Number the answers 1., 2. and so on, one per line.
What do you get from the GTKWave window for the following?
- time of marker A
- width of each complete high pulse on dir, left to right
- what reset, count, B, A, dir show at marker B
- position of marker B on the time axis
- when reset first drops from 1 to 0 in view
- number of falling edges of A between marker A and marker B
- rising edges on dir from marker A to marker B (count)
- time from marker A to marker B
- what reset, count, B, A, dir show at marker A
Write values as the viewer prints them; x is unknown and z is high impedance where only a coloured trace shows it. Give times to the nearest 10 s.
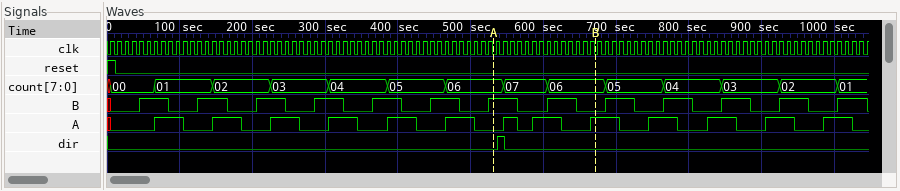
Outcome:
1. 530 s
2. 10 s
3. reset=0, count=06, B=0, A=1, dir=0
4. 670 s
5. 10 s
6. 2
7. 1
8. 140 s
9. reset=0, count=06, B=1, A=0, dir=0
